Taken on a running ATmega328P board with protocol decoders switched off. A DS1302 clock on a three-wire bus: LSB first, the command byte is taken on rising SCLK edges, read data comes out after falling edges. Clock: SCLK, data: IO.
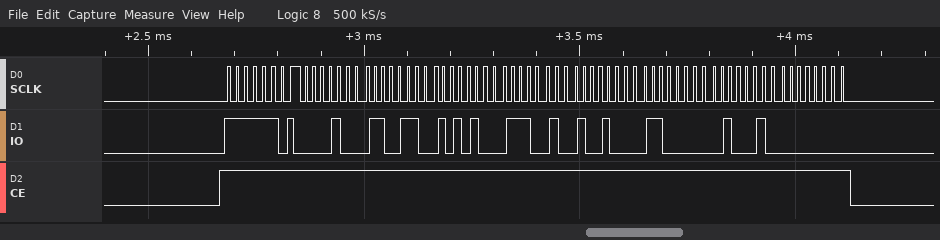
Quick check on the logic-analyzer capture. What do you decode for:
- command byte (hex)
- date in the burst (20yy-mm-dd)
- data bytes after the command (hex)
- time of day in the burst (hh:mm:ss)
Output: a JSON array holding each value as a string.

["0xBF", "2022-09-27", "10 33 15 27 09 03 22 00", "15:33:10"]
